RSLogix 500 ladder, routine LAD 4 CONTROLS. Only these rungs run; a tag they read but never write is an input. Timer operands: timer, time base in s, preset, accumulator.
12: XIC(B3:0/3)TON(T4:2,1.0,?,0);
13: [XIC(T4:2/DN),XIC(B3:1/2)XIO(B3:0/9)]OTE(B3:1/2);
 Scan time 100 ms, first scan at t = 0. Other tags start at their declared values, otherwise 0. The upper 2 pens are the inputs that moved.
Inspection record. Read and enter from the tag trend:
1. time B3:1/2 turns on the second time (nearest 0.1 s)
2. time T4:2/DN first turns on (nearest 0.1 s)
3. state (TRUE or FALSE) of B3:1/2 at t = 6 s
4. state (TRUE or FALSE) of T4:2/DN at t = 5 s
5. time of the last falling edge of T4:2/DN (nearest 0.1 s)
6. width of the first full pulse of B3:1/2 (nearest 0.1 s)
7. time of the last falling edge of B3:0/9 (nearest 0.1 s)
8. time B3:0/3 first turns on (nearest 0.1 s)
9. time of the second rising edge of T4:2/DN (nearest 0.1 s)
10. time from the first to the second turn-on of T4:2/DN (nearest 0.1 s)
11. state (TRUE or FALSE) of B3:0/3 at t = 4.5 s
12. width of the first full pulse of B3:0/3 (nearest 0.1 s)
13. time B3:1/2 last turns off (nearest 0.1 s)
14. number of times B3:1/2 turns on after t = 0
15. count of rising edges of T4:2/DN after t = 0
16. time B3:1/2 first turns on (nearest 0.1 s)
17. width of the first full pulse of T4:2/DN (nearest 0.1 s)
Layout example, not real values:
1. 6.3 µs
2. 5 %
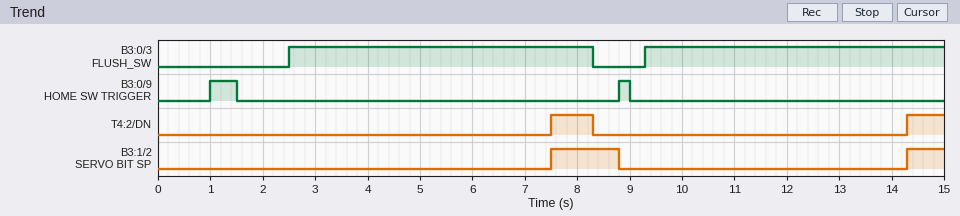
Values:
1. 14.3 s
2. 7.5 s
3. FALSE
4. FALSE
5. 8.3 s
6. 1.3 s
7. 9.0 s
8. 2.5 s
9. 14.3 s
10. 6.8 s
11. TRUE
12. 5.8 s
13. 8.8 s
14. 2
15. 2
16. 7.5 s
17. 0.8 s
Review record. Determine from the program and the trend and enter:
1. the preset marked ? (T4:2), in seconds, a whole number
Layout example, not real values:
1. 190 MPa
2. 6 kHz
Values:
1. 5 s
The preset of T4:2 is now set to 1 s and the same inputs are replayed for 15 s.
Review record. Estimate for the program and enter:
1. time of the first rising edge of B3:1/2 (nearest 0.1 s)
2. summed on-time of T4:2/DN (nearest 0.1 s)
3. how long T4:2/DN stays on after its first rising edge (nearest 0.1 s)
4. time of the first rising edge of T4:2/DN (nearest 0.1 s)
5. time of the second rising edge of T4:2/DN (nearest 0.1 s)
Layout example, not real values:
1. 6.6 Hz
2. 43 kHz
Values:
1. 3.5 s
2. 9.5 s
3. 4.8 s
4. 3.5 s
5. 10.3 s
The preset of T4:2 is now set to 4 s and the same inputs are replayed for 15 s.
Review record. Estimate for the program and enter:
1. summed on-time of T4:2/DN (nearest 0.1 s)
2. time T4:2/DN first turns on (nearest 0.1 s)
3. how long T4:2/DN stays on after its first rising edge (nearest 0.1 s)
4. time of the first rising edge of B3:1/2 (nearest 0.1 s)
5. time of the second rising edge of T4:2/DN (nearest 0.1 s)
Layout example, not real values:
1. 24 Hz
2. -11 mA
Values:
1. 3.5 s
2. 6.5 s
3. 1.8 s
4. 6.5 s
5. 13.3 s
